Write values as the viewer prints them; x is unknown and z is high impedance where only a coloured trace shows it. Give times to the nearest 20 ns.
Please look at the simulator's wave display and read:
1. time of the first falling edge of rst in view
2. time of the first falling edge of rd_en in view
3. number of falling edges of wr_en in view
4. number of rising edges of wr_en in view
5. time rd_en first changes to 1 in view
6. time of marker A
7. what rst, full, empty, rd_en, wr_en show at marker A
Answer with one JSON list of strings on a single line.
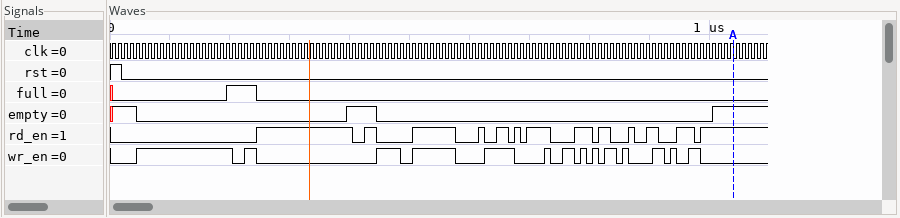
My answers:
["20 ns", "400 ns", "14", "14", "240 ns", "1040 ns", "rst=0, full=0, empty=1, rd_en=1, wr_en=0"]
